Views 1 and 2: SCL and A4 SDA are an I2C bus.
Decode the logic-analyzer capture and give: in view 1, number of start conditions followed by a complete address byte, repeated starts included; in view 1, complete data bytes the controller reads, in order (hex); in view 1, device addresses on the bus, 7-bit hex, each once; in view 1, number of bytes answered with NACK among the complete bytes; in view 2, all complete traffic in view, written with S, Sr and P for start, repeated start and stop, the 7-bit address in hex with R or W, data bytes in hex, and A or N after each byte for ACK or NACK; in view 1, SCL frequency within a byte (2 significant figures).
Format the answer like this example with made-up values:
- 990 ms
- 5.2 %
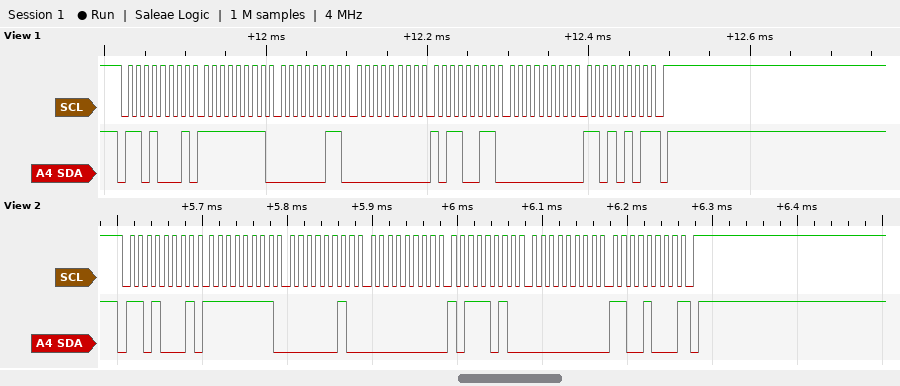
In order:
- 1
- FF 03 00 B3 00 D5
- 0x68
- 1
- S 68R A FF A 02 A 00 A BA A 00 A C8 N P
- 100 kHz
